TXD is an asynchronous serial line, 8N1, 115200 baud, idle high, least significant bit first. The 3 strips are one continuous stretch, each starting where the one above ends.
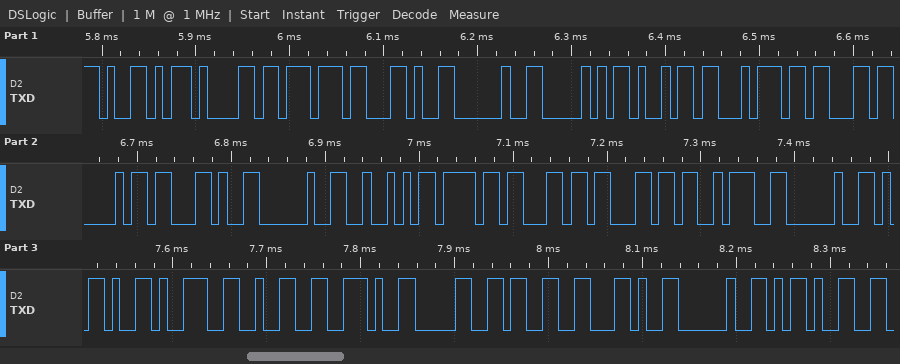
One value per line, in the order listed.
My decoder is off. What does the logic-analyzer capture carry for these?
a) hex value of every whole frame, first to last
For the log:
59 61 77 2C 20 50 69 74 63 68 2C 20 52 6F 6C 6C 3A 20 2D 39 32 2E 30 33 2C 20 2D
